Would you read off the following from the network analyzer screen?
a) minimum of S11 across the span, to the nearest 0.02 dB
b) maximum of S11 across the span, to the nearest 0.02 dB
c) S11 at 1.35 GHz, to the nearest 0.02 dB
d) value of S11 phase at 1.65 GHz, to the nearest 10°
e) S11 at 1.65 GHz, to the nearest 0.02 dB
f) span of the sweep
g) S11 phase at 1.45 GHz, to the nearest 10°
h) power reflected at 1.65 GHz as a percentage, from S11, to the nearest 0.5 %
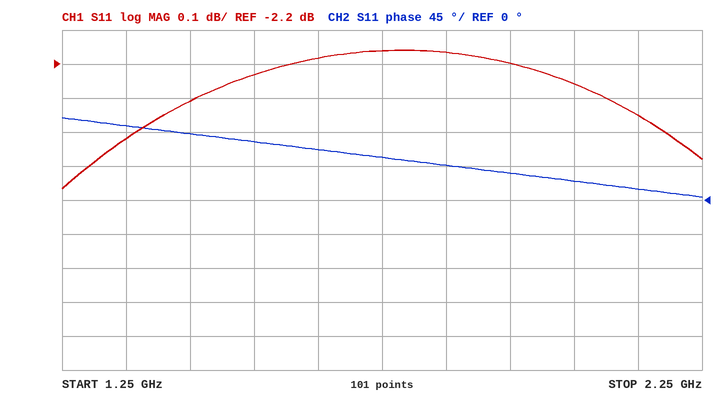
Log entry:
-2.56 dB
-2.16 dB
-2.42 dB
70°
-2.18 dB
1 GHz
90°
60.5 %
